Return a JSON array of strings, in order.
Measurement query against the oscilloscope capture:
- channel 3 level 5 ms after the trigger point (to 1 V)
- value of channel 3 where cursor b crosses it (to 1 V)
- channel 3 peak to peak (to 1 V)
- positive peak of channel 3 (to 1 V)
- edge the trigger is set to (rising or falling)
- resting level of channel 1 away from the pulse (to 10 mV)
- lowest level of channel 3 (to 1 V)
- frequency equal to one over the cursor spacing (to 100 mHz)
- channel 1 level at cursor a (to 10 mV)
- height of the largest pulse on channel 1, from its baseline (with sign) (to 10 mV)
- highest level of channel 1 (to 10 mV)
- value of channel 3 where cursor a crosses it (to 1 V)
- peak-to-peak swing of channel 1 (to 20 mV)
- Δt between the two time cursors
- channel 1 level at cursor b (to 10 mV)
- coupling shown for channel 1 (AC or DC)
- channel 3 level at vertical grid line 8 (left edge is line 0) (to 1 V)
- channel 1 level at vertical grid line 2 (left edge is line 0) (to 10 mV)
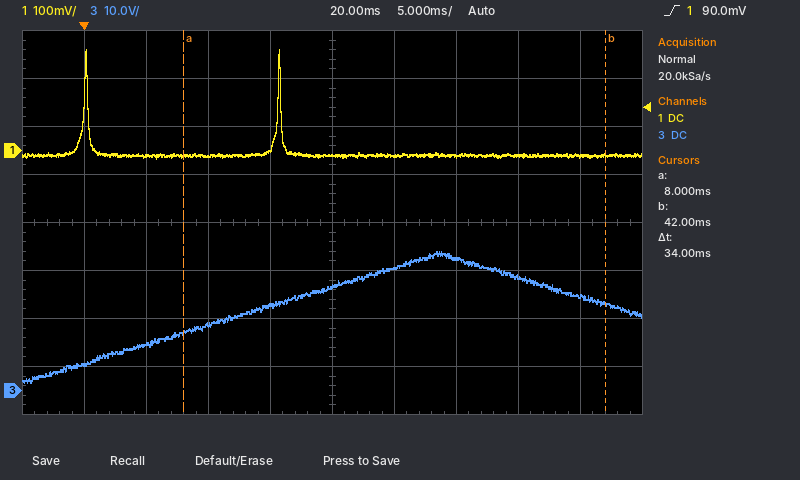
["10 V", "18 V", "27 V", "29 V", "rising", "-10 mV", "2 V", "29.4 Hz", "-10 mV", "+220 mV", "210 mV", "12 V", "220 mV", "34 ms", "-10 mV", "DC", "24 V", "-10 mV"]
